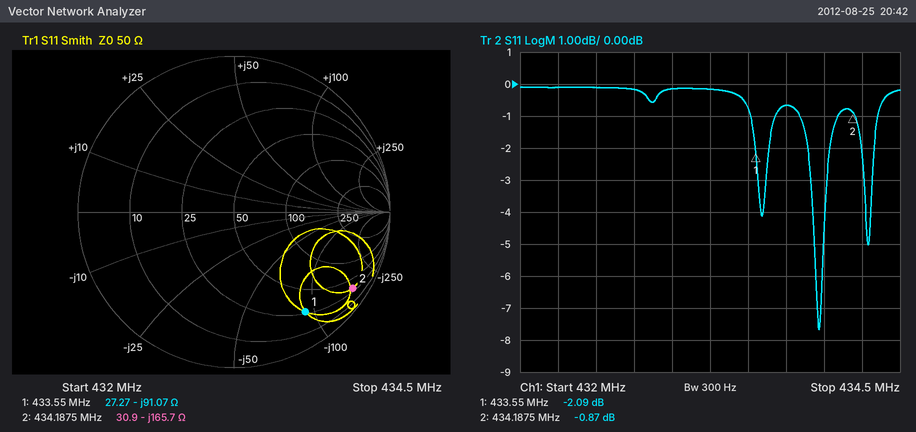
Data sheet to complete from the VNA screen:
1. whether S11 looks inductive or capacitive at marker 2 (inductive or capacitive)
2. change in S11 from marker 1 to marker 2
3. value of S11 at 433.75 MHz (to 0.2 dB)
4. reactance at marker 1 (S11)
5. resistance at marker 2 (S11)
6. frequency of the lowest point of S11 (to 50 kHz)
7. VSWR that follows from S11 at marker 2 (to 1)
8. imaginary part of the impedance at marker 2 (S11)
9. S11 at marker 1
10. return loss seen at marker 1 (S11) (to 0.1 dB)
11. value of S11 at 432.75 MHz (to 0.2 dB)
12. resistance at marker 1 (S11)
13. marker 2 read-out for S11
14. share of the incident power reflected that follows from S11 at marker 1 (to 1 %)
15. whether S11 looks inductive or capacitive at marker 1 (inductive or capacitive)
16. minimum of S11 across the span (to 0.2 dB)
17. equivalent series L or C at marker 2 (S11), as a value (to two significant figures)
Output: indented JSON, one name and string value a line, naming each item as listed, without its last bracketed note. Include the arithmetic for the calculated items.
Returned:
{
  "whether S11 looks inductive or capacitive at marker 2": "capacitive",
  "change in S11 from marker 1 to marker 2": "-0.87 − (-2.09) = 1.22 dB",
  "value of S11 at 433.75 MHz": "-0.6 dB",
  "reactance at marker 1": "-91.07 Ω",
  "resistance at marker 2": "30.9 Ω",
  "frequency of the lowest point of S11": "433.95 MHz",
  "VSWR that follows from S11 at marker 2": "(1 + 0.9047)/(1 − 0.9047) ≈ 20",
  "imaginary part of the impedance at marker 2": "-165.7 Ω",
  "S11 at marker 1": "-2.09 dB",
  "return loss seen at marker 1 (S11)": "2.1 dB",
  "value of S11 at 432.75 MHz": "-0.2 dB",
  "resistance at marker 1": "27.27 Ω",
  "marker 2 read-out for S11": "-0.87 dB",
  "share of the incident power reflected that follows from S11 at marker 1": "10^(-2.09/10) ≈ 62 %",
  "whether S11 looks inductive or capacitive at marker 1": "capacitive",
  "minimum of S11 across the span": "-7.6 dB",
  "equivalent series L or C at marker 2 (S11), as a value": "C = 1/(2π × 434.1875 MHz × 165.7 Ω) ≈ 2.2 pF"
}
